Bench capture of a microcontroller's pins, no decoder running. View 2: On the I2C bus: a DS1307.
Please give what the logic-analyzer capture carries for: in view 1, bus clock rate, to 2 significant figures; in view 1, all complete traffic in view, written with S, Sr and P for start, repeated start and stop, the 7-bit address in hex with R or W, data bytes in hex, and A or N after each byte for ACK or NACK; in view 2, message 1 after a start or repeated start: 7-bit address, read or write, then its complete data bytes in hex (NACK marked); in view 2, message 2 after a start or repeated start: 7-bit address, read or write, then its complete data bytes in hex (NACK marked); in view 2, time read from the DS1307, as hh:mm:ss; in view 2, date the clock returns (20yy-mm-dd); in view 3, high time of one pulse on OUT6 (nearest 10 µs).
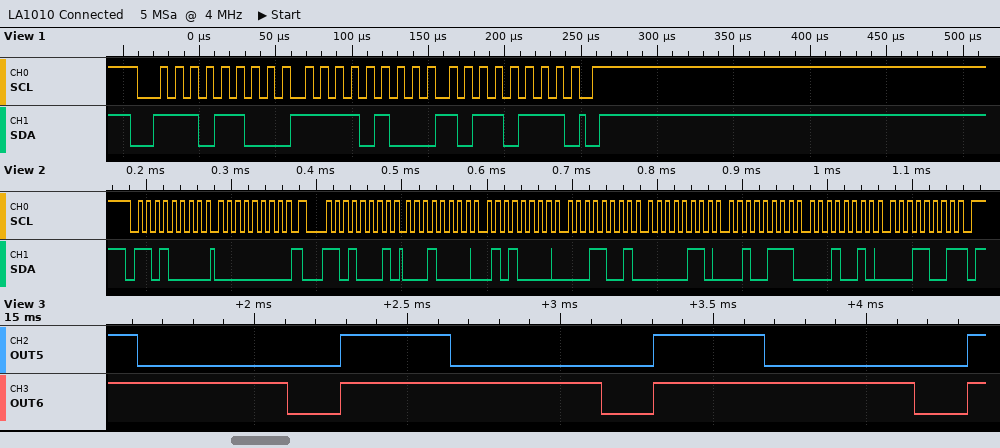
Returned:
100 kHz
S 76W A F4 A B7 A P
0x68 write: 00
0x68 read: 10 50 19 06 27 12 19 NACK
19:50:10
2019-12-27
850 µs
